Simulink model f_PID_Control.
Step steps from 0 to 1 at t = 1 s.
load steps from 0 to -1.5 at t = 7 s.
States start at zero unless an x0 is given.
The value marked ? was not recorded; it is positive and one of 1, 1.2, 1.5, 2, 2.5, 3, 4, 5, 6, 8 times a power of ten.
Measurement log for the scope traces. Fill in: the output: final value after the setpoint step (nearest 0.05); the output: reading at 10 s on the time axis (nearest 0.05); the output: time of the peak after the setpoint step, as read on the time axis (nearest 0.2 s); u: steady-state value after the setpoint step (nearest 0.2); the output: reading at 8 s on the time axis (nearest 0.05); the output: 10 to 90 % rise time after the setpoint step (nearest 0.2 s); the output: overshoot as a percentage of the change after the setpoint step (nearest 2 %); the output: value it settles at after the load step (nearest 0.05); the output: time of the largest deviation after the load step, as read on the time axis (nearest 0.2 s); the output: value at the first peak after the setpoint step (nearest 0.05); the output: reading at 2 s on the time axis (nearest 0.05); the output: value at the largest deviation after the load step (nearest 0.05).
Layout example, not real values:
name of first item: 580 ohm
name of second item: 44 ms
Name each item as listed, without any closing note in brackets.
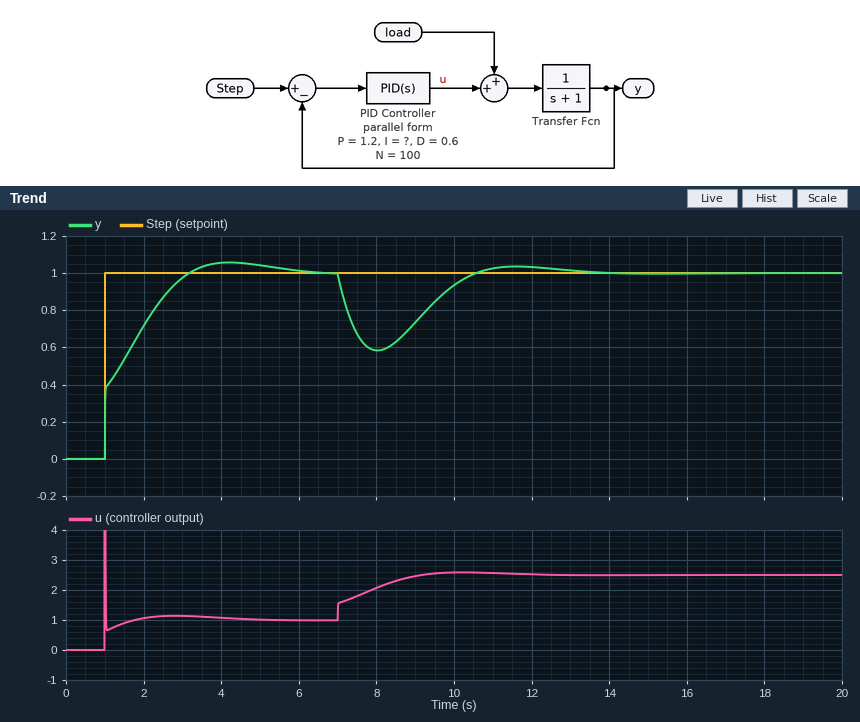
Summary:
the output: final value after the setpoint step: 1.00
the output: reading at 10 s on the time axis: 0.95
the output: time of the peak after the setpoint step, as read on the time axis: 4.2 s
u: steady-state value after the setpoint step: 1.0
the output: reading at 8 s on the time axis: 0.60
the output: 10 to 90 % rise time after the setpoint step: 1.6 s
the output: overshoot as a percentage of the change after the setpoint step: 6 %
the output: value it settles at after the load step: 1.00
the output: time of the largest deviation after the load step, as read on the time axis: 8.0 s
the output: value at the first peak after the setpoint step: 1.05
the output: reading at 2 s on the time axis: 0.70
the output: value at the largest deviation after the load step: 0.60
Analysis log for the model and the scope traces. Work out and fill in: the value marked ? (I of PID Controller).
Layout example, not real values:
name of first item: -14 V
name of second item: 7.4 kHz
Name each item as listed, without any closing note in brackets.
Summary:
the value marked ?: 2
